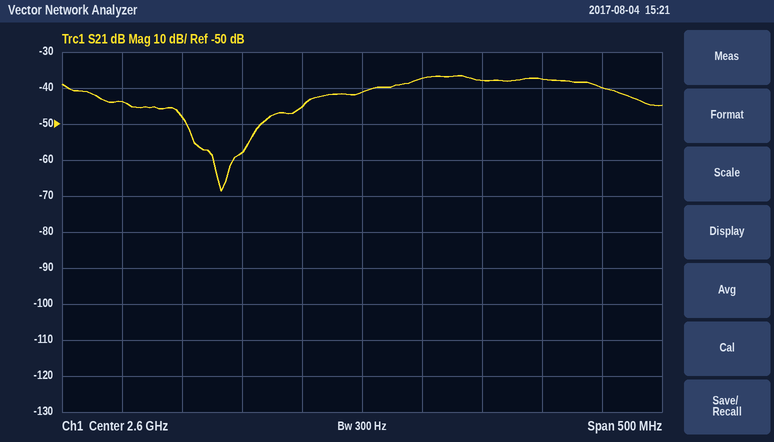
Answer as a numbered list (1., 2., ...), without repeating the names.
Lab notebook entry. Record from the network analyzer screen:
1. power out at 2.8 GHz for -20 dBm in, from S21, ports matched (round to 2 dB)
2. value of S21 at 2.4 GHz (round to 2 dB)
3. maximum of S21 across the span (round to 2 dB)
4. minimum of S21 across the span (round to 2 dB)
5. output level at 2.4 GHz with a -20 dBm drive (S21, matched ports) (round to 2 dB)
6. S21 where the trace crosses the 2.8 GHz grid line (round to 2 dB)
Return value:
1. -60 dBm
2. -44 dB
3. -36 dB
4. -68 dB
5. -64 dBm
6. -40 dB
